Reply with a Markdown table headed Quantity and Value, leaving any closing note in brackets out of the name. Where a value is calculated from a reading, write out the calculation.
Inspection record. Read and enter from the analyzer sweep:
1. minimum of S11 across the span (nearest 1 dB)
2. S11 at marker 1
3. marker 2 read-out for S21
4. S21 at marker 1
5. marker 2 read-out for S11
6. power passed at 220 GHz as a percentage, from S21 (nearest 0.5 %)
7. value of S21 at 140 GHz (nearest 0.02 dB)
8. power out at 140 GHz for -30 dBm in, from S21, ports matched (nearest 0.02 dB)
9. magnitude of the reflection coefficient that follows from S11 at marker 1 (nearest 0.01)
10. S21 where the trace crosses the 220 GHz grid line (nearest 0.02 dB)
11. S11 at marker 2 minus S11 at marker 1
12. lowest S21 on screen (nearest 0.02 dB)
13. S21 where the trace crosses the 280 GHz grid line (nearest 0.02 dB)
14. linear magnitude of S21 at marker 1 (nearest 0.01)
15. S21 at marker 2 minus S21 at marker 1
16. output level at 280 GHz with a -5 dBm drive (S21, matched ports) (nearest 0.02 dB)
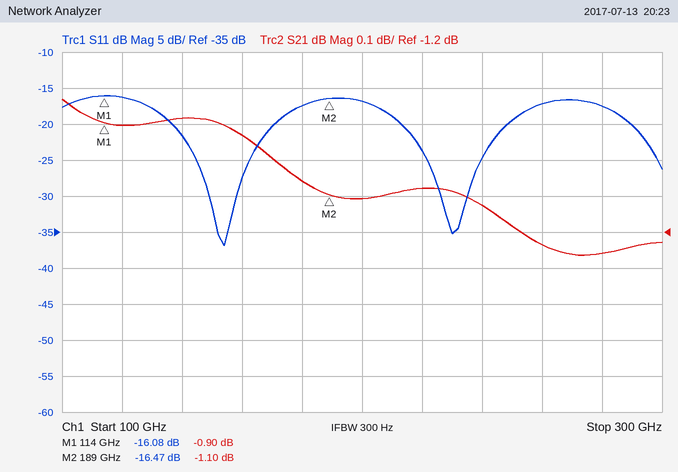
| Quantity | Value |
|---|---|
| minimum of S11 across the span | -37 dB |
| S11 at marker 1 | -16.08 dB |
| marker 2 read-out for S21 | -1.10 dB |
| S21 at marker 1 | -0.90 dB |
| marker 2 read-out for S11 | -16.47 dB |
| power passed at 220 GHz as a percentage, from S21 | 10^(-1.08/10) ≈ 78.0 % |
| value of S21 at 140 GHz | -0.88 dB |
| power out at 140 GHz for -30 dBm in, from S21, ports matched | -30 dBm + (-0.88 dB) = -30.88 dBm |
| magnitude of the reflection coefficient that follows from S11 at marker 1 | 10^(-16.08/20) ≈ 0.16 |
| S21 where the trace crosses the 220 GHz grid line | -1.08 dB |
| S11 at marker 2 minus S11 at marker 1 | -16.47 − (-16.08) = -0.39 dB |
| lowest S21 on screen | -1.26 dB |
| S21 where the trace crosses the 280 GHz grid line | -1.26 dB |
| linear magnitude of S21 at marker 1 | 10^(-0.9/20) ≈ 0.90 |
| S21 at marker 2 minus S21 at marker 1 | -1.1 − (-0.9) = -0.20 dB |
| output level at 280 GHz with a -5 dBm drive (S21, matched ports) | -5 dBm + (-1.26 dB) = -6.26 dBm |
